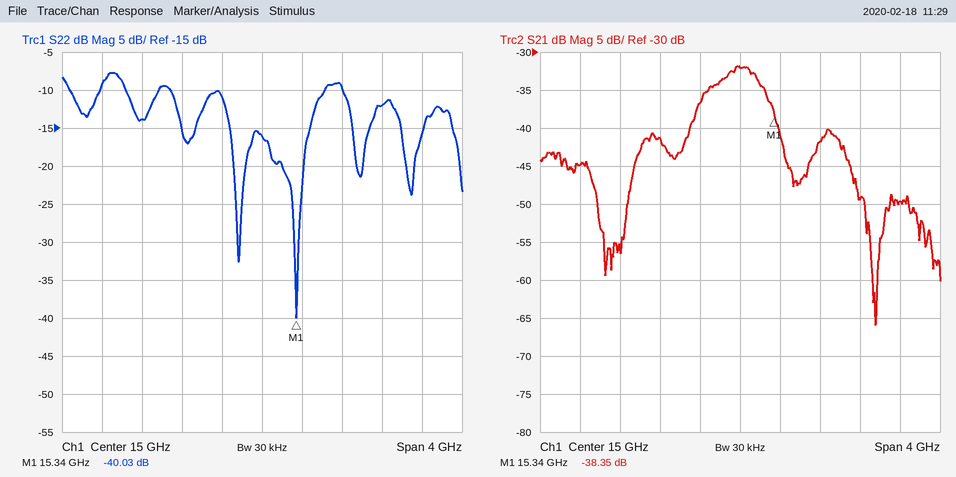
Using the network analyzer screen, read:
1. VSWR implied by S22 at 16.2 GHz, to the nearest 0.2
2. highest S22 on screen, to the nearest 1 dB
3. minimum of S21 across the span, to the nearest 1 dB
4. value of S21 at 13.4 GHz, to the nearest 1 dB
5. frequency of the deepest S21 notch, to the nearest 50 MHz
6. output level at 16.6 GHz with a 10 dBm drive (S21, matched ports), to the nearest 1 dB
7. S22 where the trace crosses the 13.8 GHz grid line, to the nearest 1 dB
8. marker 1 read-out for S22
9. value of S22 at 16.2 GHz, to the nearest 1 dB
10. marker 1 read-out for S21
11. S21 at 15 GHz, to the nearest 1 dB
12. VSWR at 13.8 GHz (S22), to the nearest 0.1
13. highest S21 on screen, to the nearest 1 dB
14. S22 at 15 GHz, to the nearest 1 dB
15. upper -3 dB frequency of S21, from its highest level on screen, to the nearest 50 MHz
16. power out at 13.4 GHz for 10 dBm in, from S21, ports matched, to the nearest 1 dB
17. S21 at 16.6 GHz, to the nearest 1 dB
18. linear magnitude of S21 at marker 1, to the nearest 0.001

1.6
-8 dB
-66 dB
-45 dB
16.35 GHz
-40 dBm
-14 dB
-40.03 dB
-12 dB
-38.35 dB
-32 dB
1.5
-32 dB
-16 dB
15.25 GHz
-35 dBm
-50 dB
0.012
